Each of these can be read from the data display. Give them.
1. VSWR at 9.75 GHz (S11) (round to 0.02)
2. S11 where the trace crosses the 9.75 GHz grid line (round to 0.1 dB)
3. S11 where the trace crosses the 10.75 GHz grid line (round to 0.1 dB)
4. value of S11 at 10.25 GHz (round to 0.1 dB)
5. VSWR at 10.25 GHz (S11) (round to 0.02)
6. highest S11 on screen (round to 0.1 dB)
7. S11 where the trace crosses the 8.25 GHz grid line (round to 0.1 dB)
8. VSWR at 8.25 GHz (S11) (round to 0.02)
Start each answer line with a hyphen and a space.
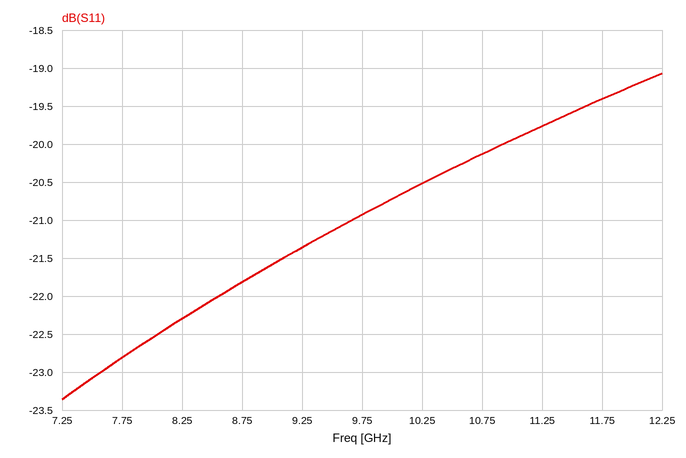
- 1.20
- -20.9 dB
- -20.1 dB
- -20.5 dB
- 1.20
- -19.1 dB
- -22.3 dB
- 1.16
